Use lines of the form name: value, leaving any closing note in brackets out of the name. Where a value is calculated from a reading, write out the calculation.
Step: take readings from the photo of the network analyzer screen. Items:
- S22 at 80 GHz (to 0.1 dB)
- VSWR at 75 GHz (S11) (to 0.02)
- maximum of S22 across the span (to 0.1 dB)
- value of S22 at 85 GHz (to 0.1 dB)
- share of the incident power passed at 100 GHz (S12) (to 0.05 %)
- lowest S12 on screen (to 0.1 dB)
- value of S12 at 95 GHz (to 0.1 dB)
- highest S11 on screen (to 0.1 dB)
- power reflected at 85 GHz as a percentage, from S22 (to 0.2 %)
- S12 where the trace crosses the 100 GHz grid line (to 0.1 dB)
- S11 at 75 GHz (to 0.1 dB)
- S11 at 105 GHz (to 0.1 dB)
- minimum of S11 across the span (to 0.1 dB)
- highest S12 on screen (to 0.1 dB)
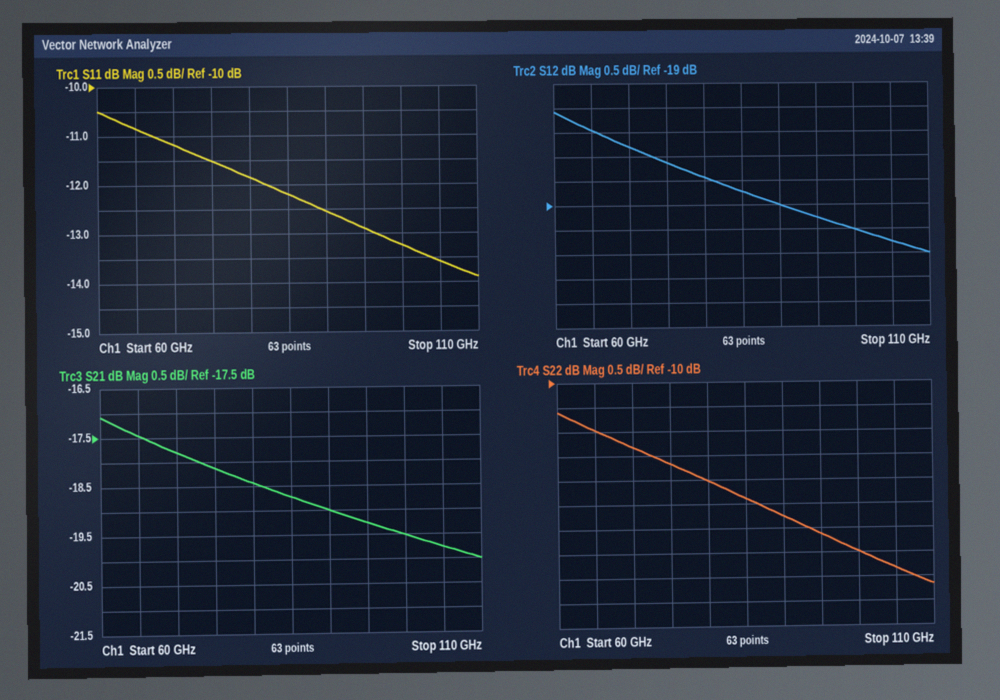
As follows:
S22 at 80 GHz: -12.0 dB
VSWR at 75 GHz (S11): |Γ| = 10^(-11.5/20) = 0.2661; VSWR = (1 + 0.2661)/(1 − 0.2661) ≈ 1.73, so 1.72 to the nearest 0.02
maximum of S22 across the span: -10.6 dB
value of S22 at 85 GHz: -12.4 dB
share of the incident power passed at 100 GHz (S12): 10^(-19.5/10) ≈ 1.12 %, so 1.10 % to the nearest 0.05 %
lowest S12 on screen: -20.0 dB
value of S12 at 95 GHz: -19.3 dB
highest S11 on screen: -10.5 dB
power reflected at 85 GHz as a percentage, from S22: 10^(-12.4/10) ≈ 5.8 %
S12 where the trace crosses the 100 GHz grid line: -19.5 dB
S11 at 75 GHz: -11.5 dB
S11 at 105 GHz: -13.6 dB
minimum of S11 across the span: -13.9 dB
highest S12 on screen: -17.1 dB
